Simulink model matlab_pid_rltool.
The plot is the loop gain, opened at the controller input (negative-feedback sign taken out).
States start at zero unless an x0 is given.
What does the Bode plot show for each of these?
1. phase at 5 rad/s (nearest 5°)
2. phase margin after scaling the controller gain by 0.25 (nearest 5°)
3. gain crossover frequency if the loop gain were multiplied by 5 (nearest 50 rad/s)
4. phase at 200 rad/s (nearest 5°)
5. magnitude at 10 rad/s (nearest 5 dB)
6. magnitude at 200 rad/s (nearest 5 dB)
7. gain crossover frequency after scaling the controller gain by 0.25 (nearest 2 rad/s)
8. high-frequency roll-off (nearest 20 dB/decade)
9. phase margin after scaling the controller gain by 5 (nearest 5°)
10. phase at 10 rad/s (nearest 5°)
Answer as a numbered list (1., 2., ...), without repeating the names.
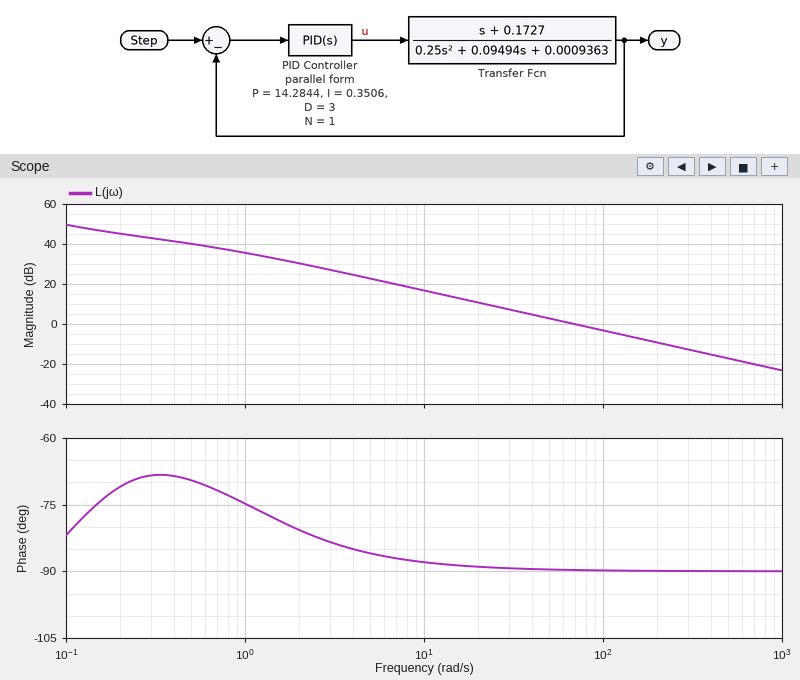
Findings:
1. -85°
2. 90°
3. 350 rad/s
4. -90°
5. 15 dB
6. -10 dB
7. 18 rad/s
8. -20 dB/decade
9. 90°
10. -90°
